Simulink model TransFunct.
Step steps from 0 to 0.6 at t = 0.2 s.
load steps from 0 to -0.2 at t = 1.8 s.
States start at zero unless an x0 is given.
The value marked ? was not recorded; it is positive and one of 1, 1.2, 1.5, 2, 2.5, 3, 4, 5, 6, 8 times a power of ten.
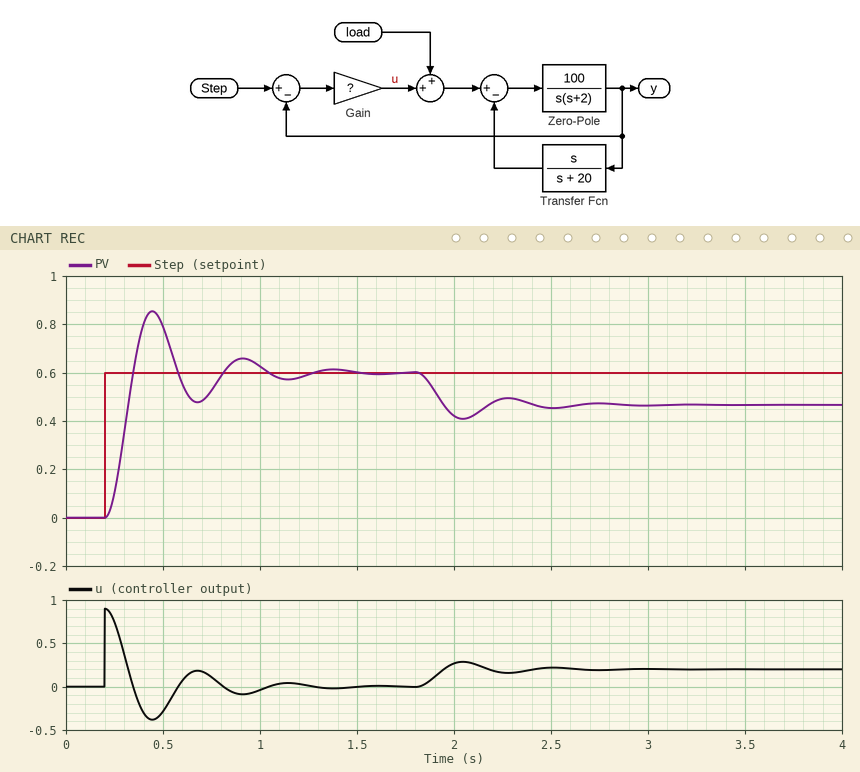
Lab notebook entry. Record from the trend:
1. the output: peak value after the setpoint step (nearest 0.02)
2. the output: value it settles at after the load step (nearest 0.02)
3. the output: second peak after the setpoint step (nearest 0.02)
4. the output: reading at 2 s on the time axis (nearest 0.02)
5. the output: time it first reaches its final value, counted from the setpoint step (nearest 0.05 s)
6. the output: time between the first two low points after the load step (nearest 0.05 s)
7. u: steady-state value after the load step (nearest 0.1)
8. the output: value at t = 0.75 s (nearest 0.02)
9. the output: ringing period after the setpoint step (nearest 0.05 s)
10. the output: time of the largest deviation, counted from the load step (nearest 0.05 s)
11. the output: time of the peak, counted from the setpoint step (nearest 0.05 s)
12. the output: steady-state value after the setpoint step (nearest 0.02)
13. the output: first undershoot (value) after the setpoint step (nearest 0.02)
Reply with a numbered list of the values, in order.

1. 0.86
2. 0.46
3. 0.66
4. 0.42
5. 0.15 s
6. 0.45 s
7. 0.2
8. 0.52
9. 0.45 s
10. 0.25 s
11. 0.25 s
12. 0.60
13. 0.48
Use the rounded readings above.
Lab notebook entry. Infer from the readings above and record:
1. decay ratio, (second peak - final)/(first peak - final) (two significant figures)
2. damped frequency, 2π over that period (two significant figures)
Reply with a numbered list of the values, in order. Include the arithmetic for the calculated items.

1. (0.66 - 0.6) / (0.86 - 0.6) = 0.23
2. 2π / 0.45 = 14 rad/s
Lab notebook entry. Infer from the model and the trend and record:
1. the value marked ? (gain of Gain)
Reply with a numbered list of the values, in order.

1. 1.5
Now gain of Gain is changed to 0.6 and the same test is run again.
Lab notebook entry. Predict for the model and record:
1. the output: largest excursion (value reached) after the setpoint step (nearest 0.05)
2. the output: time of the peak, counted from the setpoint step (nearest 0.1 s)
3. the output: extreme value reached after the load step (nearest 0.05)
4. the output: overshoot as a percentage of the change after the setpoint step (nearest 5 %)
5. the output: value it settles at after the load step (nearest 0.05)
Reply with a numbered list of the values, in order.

1. 0.70
2. 0.4 s
3. 0.20
4. 20 %
5. 0.25
